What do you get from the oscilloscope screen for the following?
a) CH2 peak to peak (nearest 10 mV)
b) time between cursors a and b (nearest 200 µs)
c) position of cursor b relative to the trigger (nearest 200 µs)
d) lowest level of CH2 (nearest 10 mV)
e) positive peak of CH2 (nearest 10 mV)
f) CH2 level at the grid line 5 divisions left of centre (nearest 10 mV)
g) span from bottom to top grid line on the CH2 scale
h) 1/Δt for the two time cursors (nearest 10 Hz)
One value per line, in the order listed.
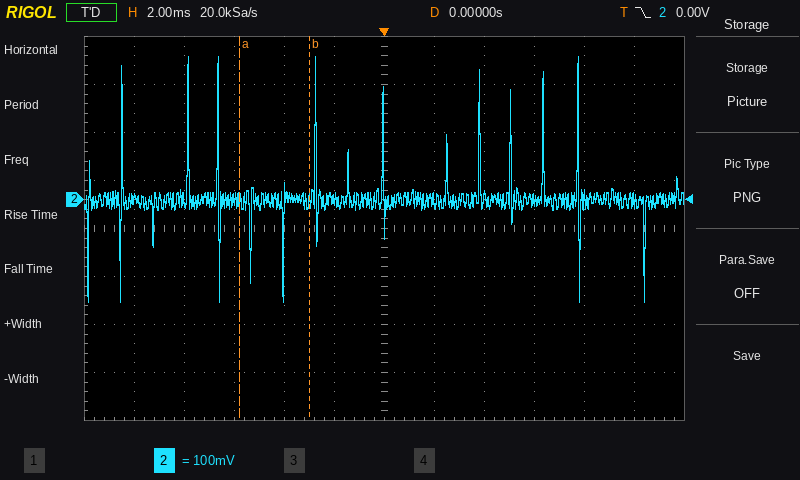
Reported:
510 mV
2.8 ms
-3.0 ms
-210 mV
300 mV
0 mV
800 mV
360 Hz
